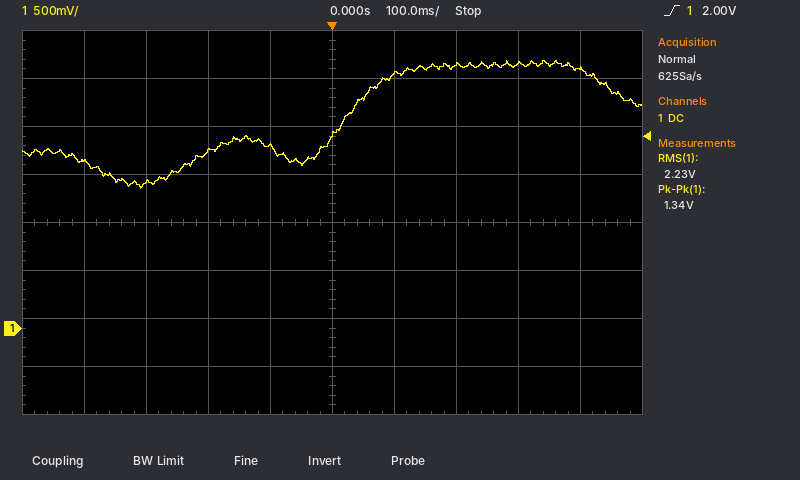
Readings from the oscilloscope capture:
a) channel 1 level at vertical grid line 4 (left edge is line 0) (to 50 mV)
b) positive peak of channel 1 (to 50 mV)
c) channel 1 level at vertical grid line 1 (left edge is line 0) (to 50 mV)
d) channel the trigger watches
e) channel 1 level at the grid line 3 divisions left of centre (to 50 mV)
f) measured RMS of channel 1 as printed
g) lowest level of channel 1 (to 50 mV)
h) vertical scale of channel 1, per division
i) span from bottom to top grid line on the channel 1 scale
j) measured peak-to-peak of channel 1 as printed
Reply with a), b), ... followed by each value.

a) 1.90 V
b) 2.80 V
c) 1.75 V
d) channel 1
e) 1.50 V
f) 2.23 V
g) 1.45 V
h) 500 mV
i) 4 V
j) 1.34 V
